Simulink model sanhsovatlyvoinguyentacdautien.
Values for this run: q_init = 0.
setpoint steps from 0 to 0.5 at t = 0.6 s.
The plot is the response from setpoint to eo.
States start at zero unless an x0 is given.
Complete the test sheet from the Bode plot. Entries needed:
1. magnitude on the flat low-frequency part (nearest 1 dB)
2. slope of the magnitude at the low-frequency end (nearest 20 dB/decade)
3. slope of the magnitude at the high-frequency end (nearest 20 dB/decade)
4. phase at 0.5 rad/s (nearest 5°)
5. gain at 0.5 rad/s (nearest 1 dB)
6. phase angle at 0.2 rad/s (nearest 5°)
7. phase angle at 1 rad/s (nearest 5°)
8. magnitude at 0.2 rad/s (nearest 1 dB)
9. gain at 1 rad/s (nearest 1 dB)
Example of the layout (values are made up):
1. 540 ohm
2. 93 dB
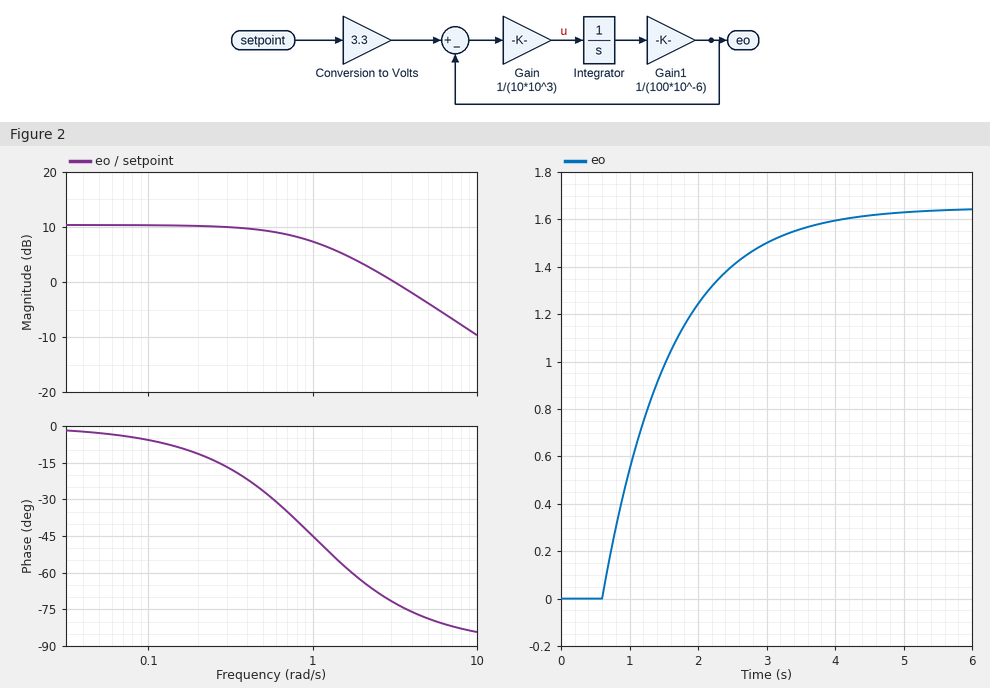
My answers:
1. 10 dB
2. 0 dB/decade
3. -20 dB/decade
4. -25°
5. 9 dB
6. -10°
7. -45°
8. 10 dB
9. 7 dB
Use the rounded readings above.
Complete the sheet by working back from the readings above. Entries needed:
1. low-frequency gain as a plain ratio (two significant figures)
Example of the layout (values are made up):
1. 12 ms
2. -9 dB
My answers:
1. 3.2
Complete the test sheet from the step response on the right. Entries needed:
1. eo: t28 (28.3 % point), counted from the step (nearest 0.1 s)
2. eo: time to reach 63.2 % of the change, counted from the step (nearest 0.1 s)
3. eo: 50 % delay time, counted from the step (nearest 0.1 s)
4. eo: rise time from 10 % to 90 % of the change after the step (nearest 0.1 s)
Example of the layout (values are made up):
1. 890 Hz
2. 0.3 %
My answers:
1. 0.3 s
2. 1.0 s
3. 0.7 s
4. 2.2 s
